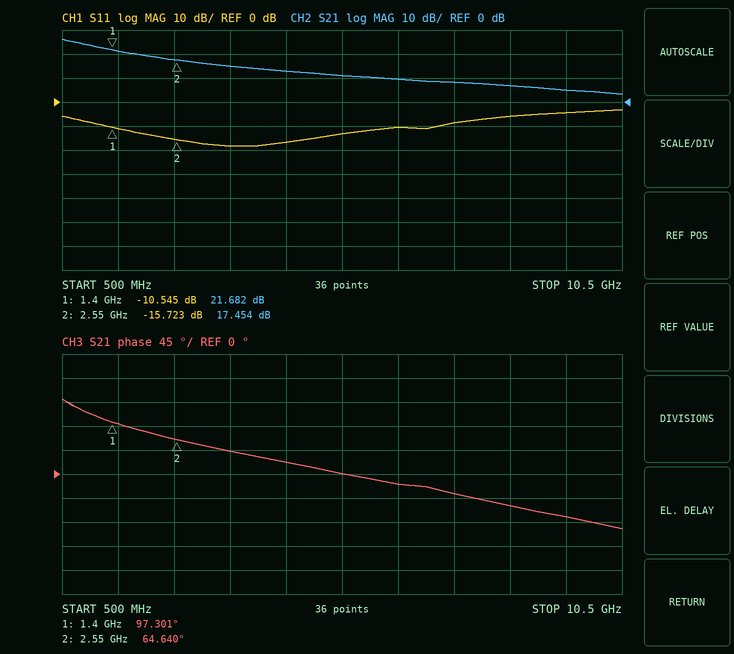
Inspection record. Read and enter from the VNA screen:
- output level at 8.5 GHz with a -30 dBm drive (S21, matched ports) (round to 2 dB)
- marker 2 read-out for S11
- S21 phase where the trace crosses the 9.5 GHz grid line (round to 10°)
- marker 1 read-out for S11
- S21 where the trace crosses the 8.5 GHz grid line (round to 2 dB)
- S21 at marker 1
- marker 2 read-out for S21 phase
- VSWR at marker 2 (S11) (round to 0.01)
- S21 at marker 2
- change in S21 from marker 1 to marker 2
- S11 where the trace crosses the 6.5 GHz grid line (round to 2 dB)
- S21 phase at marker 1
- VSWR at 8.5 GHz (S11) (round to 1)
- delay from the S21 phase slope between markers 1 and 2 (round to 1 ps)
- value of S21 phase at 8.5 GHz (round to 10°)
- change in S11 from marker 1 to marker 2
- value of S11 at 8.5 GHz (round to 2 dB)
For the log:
-24 dBm
-15.723 dB
-80°
-10.545 dB
6 dB
21.682 dB
64.640°
1.39
17.454 dB
-4.228 dB
-10 dB
97.301°
3
79 ps
-60°
-5.178 dB
-6 dB
